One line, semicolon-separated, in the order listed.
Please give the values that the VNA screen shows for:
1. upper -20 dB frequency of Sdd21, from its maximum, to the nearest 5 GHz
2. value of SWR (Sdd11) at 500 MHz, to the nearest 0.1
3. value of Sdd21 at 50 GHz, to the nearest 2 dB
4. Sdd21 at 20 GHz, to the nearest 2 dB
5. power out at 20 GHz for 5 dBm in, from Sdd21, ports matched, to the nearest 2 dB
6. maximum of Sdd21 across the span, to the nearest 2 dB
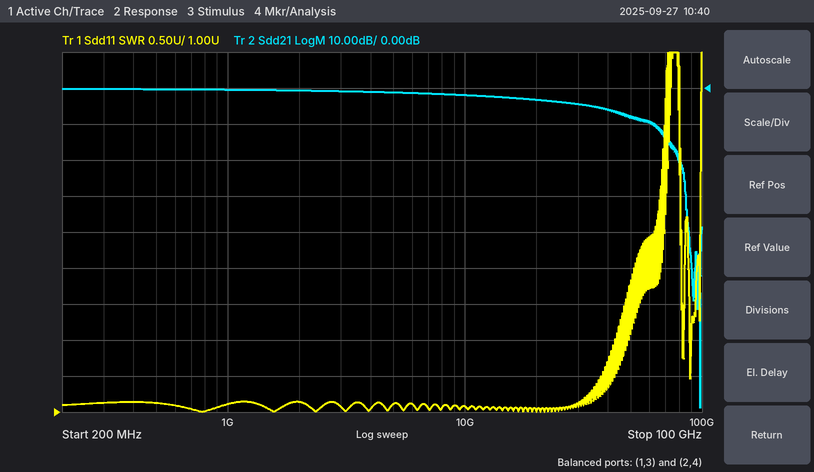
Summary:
80 GHz; 1.1; -8 dB; -4 dB; 2 dBm; 0 dB
